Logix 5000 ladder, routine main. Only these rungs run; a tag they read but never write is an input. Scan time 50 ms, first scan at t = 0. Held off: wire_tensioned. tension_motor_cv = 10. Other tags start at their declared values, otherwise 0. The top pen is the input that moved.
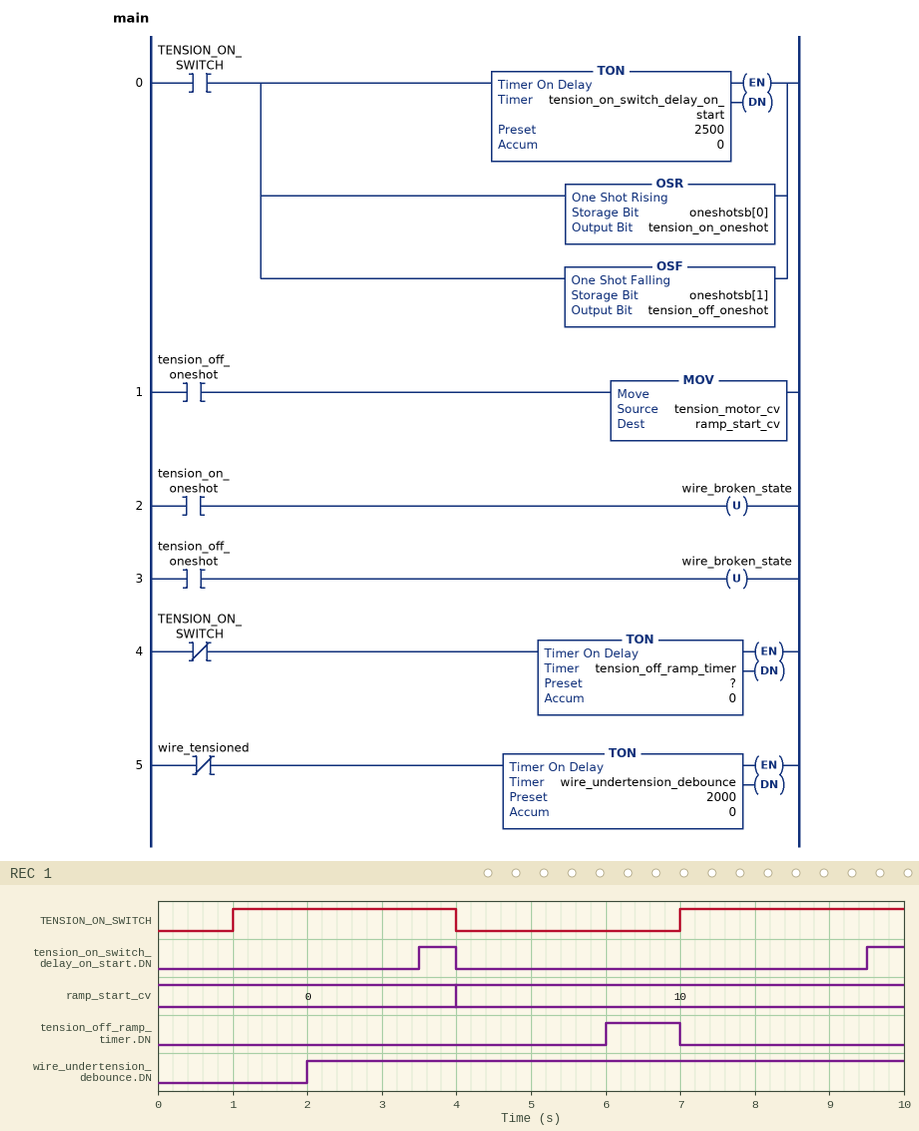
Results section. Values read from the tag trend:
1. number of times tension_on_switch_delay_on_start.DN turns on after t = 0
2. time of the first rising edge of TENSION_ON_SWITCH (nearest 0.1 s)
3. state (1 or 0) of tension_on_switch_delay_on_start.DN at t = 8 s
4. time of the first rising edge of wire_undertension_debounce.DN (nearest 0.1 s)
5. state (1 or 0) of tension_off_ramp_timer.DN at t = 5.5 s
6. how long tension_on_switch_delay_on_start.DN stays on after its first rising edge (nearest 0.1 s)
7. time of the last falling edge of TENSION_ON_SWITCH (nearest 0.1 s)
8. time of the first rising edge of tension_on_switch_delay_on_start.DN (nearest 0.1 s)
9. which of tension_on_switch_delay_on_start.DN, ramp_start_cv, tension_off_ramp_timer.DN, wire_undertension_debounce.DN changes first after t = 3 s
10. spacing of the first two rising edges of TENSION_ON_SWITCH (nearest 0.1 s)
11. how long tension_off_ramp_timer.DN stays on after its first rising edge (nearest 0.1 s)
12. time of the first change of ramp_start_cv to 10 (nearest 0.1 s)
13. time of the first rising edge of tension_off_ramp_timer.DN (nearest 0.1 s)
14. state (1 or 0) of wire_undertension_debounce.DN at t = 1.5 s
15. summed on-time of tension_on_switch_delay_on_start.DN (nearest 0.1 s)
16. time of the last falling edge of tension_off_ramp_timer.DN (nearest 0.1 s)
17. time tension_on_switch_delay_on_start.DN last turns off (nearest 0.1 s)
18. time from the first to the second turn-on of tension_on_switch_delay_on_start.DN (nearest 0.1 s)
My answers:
2
1.0 s
0
2.0 s
0
0.5 s
4.0 s
3.5 s
tension_on_switch_delay_on_start.DN
6.0 s
1.0 s
4.0 s
6.0 s
0
1.0 s
7.0 s
4.0 s
6.0 s
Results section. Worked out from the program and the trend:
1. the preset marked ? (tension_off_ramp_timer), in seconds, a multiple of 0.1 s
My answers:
2.0 s
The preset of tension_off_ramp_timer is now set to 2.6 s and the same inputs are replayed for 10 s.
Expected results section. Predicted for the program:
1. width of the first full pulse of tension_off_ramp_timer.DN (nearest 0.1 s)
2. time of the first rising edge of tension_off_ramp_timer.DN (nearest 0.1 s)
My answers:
0.4 s
6.6 s
